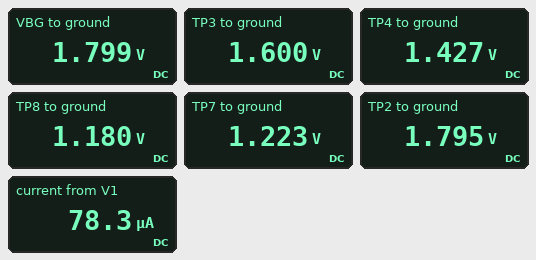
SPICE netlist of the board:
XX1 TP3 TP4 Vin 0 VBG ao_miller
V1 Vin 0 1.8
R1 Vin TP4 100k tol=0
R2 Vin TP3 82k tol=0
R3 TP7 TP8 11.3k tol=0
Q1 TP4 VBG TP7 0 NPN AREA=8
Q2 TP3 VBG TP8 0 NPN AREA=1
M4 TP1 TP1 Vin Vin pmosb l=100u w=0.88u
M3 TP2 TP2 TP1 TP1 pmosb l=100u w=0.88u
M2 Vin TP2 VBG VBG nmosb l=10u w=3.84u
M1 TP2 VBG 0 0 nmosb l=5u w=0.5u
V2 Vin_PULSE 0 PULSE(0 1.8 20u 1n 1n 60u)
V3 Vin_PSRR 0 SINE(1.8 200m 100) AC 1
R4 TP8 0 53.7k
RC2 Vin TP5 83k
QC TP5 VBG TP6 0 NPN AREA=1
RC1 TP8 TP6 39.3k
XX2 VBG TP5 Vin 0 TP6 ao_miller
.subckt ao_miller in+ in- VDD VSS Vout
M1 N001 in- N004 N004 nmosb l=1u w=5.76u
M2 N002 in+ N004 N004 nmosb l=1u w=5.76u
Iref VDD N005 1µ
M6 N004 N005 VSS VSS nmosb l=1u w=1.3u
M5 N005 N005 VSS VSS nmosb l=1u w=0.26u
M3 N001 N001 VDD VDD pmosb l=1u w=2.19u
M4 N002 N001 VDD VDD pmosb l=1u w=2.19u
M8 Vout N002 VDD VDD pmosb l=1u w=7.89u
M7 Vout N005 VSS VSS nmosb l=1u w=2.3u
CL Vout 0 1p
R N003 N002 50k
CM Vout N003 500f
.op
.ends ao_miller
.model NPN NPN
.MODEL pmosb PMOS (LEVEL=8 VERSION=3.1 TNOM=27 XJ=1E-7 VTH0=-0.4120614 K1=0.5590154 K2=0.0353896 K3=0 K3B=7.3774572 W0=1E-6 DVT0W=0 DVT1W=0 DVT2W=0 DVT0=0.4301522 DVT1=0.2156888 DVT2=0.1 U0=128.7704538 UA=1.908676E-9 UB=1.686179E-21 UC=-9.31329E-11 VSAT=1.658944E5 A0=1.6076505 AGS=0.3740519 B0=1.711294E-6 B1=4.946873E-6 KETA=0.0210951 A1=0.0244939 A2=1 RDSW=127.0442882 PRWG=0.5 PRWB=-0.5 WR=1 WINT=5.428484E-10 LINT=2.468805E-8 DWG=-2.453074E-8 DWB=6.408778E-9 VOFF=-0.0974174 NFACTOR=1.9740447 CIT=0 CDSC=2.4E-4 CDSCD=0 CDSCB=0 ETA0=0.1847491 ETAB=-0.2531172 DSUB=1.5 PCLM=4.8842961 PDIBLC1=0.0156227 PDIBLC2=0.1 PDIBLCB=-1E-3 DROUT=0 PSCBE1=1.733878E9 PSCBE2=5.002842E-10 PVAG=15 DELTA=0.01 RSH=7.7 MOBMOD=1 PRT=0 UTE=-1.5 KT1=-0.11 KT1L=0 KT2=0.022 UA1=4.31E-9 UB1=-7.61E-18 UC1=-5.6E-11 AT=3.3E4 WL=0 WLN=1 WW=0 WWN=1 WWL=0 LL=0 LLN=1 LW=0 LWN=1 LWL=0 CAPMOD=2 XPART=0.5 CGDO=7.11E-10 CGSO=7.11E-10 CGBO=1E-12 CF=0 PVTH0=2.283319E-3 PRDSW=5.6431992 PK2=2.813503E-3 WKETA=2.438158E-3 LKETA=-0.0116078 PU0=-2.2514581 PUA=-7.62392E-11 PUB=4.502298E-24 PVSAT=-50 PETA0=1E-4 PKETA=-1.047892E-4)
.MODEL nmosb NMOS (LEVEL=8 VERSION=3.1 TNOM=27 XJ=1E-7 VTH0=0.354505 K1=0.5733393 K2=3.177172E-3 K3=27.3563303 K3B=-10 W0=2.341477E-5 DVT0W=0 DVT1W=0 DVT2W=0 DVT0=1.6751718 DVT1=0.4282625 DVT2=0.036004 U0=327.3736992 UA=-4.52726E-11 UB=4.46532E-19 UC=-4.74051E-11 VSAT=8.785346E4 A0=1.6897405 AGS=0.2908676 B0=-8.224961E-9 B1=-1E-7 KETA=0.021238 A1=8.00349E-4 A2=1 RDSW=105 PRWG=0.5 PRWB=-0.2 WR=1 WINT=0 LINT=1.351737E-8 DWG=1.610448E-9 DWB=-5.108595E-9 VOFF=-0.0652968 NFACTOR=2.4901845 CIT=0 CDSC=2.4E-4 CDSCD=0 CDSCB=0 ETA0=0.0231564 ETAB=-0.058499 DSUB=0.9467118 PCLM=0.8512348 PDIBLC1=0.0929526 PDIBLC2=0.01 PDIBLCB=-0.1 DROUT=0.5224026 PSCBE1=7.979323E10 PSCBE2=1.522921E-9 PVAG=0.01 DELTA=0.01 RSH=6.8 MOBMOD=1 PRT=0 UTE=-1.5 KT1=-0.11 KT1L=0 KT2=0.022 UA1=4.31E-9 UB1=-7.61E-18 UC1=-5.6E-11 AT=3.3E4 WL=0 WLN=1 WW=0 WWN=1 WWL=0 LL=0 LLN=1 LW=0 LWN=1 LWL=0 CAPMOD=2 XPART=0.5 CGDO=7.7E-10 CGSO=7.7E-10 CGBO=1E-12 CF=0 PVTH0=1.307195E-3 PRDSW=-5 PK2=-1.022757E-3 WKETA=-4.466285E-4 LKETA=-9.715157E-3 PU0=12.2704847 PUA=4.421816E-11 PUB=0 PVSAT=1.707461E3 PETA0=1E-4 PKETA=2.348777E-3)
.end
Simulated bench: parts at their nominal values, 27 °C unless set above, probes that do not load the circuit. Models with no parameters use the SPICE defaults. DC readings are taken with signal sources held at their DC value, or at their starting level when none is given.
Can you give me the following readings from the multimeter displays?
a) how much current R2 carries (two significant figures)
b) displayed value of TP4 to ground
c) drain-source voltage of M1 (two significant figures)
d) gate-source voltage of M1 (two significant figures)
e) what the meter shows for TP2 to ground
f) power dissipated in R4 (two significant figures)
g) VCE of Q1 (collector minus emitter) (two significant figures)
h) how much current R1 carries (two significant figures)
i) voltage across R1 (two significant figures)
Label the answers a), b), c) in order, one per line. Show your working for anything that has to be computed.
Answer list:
a) (1.8 V - 1.6 V) / 82 kΩ = 2.4 µA
b) 1.427 V
c) 1.795 V = 1.8 V
d) 1.799 V = 1.8 V
e) 1.795 V
f) (1.18 V)^2 / 53.7 kΩ = 26 µW
g) 1.427 V - 1.223 V = 200 mV
h) (1.8 V - 1.427 V) / 100 kΩ = 3.7 µA
i) 1.8 V - 1.427 V = 370 mV
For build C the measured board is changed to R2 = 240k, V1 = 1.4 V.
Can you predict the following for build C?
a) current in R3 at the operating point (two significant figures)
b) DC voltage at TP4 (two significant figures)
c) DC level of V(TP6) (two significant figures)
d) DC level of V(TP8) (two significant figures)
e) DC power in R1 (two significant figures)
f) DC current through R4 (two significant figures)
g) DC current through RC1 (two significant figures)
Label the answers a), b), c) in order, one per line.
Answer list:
a) 1.2 µA
b) 1.3 V
c) 1.4 V
d) 840 mV
e) 140 nW
f) 16 µA
g) 14 µA
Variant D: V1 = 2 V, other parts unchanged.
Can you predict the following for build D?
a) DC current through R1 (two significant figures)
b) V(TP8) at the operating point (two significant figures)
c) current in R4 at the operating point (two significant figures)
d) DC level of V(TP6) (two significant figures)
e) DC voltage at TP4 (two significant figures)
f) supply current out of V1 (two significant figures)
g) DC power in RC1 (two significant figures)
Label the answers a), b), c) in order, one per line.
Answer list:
a) 4.4 µA
b) 1.4 V
c) 25 µA
d) 2.0 V
e) 1.6 V
f) 89 µA
g) 10 µW
